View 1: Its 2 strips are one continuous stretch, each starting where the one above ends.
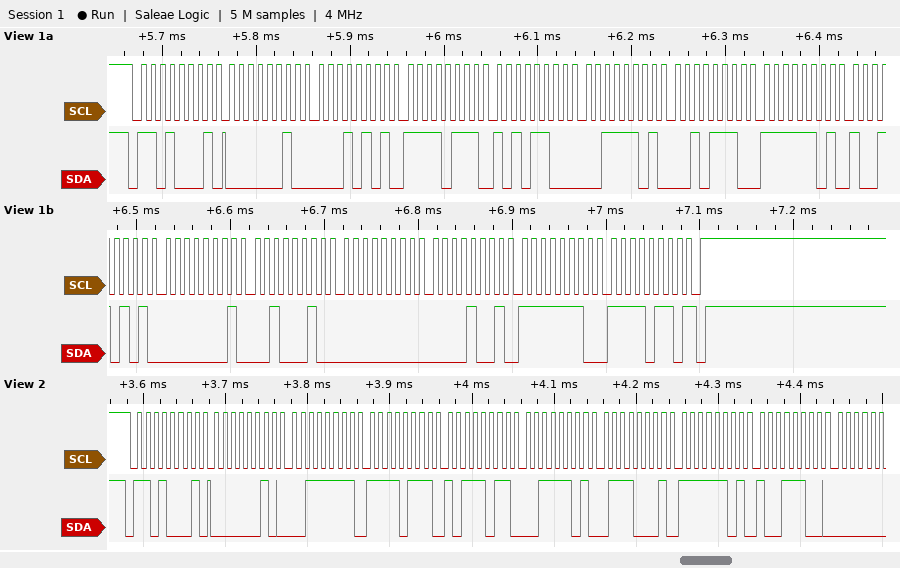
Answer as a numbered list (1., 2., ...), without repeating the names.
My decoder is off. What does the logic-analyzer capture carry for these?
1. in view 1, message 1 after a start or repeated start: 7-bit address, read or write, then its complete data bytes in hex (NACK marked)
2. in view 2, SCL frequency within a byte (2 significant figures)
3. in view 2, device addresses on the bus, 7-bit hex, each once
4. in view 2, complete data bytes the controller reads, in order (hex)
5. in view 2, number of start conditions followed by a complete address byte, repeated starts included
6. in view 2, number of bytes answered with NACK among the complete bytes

1. 0x68 read: 02 15 F7 AC 3D 2E FD 95 01 22 00 09 FE F6 NACK
2. 100 kHz
3. 0x68
4. 02 3F F7 BB 3D 71 FD 9C
5. 1
6. 0
